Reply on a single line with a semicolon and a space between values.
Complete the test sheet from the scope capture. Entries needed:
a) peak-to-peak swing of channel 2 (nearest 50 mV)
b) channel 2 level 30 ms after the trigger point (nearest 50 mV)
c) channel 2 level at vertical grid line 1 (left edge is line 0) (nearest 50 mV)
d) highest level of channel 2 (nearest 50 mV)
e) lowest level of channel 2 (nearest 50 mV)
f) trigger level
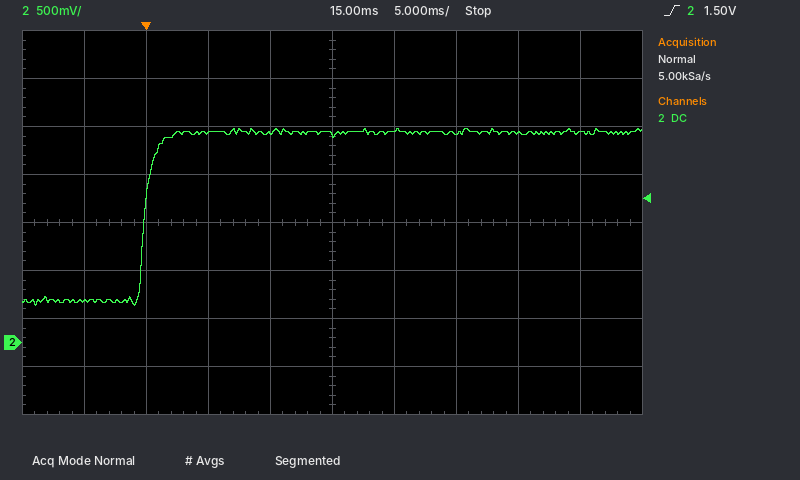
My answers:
1.85 V; 2.20 V; 450 mV; 2.25 V; 400 mV; 1.50 V
